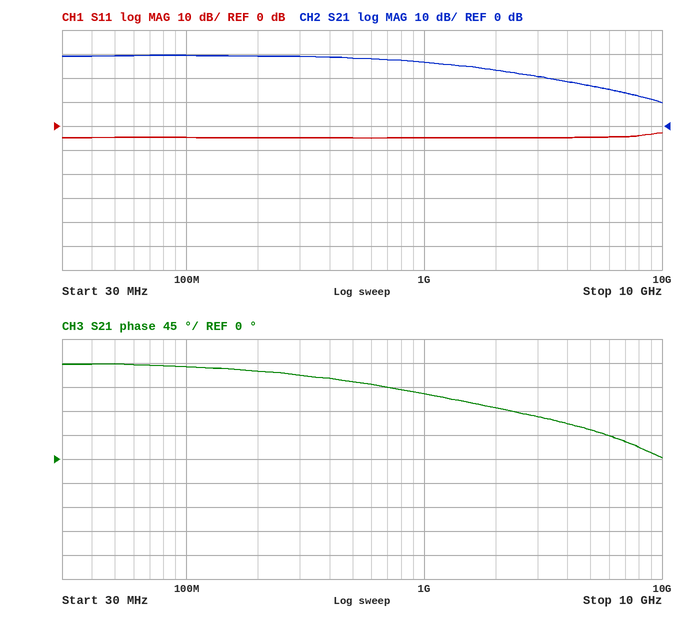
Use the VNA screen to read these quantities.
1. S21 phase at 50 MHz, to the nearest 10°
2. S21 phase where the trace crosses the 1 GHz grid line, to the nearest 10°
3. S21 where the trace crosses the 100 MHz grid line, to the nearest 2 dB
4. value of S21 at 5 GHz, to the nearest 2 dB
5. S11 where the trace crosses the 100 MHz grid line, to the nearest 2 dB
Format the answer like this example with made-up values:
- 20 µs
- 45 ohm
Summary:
- 180°
- 120°
- 30 dB
- 16 dB
- -4 dB
